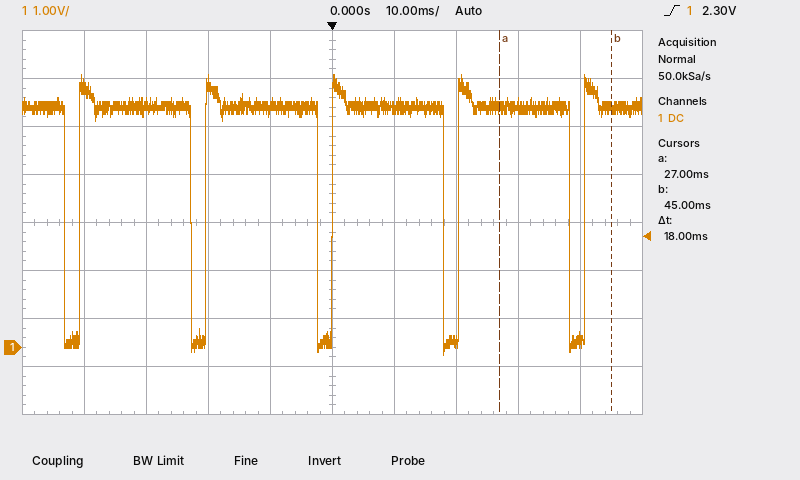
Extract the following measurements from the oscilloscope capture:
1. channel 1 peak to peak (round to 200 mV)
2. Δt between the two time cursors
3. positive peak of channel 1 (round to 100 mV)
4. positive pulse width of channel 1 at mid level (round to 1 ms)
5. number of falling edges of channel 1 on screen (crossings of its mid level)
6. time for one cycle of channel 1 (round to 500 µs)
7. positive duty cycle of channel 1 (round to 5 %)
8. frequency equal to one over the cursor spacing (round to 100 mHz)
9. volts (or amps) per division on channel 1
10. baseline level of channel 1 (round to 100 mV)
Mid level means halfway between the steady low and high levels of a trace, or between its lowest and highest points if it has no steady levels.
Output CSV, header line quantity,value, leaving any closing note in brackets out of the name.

quantity,value
channel 1 peak to peak,5.8 V
Δt between the two time cursors,18 ms
positive peak of channel 1,5.7 V
positive pulse width of channel 1 at mid level,18 ms
number of falling edges of channel 1 on screen,5
time for one cycle of channel 1,20.5 ms
positive duty cycle of channel 1,90 %
frequency equal to one over the cursor spacing,55.6 Hz
volts (or amps) per division on channel 1,1 V
baseline level of channel 1,5.0 V
